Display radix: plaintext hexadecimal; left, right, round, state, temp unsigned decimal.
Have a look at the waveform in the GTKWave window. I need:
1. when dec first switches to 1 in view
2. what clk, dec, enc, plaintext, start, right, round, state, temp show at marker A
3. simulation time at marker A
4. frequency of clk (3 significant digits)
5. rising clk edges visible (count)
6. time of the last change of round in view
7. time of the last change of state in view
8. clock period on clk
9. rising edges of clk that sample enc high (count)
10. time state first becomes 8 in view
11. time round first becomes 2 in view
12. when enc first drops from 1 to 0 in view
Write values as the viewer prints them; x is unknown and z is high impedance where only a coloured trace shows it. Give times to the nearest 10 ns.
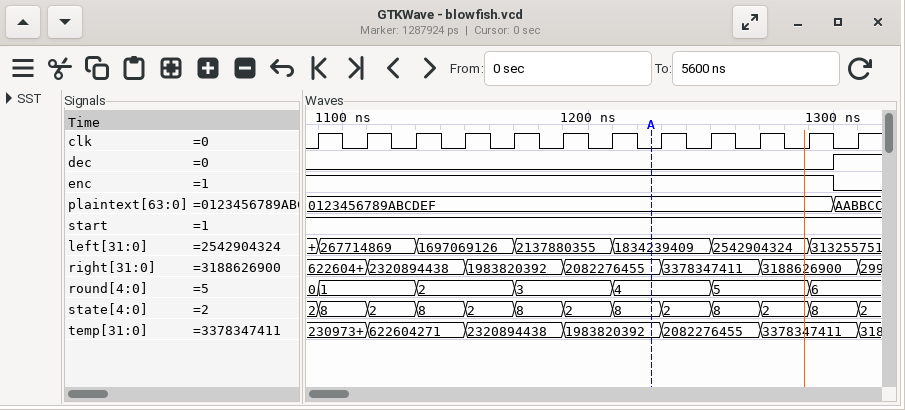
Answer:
1300 ns
clk=0, dec=0, enc=1, plaintext=0123456789ABCDEF, start=1, right=2082276455, round=4, state=8, temp=1983820392
1230 ns
50.0 MHz
12
1290 ns
1310 ns
20 ns
11
1090 ns
1130 ns
1300 ns
